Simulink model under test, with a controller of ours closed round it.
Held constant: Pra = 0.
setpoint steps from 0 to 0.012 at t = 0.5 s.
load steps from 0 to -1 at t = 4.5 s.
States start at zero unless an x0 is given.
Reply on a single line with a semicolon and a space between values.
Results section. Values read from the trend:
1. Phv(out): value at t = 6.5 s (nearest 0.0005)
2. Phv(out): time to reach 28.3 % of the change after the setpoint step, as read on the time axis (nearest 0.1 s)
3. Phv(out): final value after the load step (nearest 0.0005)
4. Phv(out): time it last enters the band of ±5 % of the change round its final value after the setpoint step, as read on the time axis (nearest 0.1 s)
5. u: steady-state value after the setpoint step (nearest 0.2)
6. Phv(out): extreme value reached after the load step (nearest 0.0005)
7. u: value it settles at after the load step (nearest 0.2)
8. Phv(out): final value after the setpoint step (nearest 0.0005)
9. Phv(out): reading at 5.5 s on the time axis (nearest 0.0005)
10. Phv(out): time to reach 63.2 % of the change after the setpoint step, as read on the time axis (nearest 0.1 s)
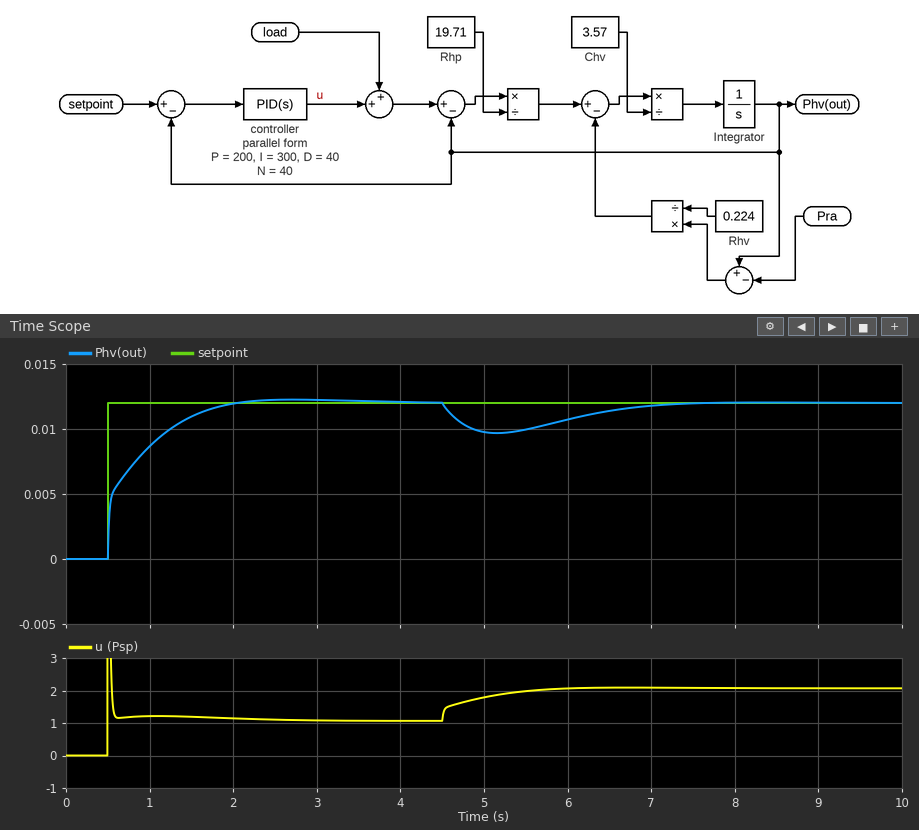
0.0115; 0.5 s; 0.0120; 1.7 s; 1.0; 0.0095; 2.0; 0.0120; 0.0100; 0.8 s
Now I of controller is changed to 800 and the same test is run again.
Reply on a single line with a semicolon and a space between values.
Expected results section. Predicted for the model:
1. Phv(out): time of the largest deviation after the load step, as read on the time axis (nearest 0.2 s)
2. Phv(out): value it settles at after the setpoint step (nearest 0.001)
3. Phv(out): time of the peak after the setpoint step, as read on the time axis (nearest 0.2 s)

5.0 s; 0.012; 1.6 s
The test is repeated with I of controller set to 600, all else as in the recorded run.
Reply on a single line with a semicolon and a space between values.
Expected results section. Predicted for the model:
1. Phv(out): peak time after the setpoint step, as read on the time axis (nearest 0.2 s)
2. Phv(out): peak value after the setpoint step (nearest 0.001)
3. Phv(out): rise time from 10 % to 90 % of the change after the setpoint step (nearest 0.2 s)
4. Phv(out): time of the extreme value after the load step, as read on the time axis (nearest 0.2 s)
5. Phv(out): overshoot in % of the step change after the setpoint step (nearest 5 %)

1.8 s; 0.013; 0.6 s; 5.0 s; 10 %
